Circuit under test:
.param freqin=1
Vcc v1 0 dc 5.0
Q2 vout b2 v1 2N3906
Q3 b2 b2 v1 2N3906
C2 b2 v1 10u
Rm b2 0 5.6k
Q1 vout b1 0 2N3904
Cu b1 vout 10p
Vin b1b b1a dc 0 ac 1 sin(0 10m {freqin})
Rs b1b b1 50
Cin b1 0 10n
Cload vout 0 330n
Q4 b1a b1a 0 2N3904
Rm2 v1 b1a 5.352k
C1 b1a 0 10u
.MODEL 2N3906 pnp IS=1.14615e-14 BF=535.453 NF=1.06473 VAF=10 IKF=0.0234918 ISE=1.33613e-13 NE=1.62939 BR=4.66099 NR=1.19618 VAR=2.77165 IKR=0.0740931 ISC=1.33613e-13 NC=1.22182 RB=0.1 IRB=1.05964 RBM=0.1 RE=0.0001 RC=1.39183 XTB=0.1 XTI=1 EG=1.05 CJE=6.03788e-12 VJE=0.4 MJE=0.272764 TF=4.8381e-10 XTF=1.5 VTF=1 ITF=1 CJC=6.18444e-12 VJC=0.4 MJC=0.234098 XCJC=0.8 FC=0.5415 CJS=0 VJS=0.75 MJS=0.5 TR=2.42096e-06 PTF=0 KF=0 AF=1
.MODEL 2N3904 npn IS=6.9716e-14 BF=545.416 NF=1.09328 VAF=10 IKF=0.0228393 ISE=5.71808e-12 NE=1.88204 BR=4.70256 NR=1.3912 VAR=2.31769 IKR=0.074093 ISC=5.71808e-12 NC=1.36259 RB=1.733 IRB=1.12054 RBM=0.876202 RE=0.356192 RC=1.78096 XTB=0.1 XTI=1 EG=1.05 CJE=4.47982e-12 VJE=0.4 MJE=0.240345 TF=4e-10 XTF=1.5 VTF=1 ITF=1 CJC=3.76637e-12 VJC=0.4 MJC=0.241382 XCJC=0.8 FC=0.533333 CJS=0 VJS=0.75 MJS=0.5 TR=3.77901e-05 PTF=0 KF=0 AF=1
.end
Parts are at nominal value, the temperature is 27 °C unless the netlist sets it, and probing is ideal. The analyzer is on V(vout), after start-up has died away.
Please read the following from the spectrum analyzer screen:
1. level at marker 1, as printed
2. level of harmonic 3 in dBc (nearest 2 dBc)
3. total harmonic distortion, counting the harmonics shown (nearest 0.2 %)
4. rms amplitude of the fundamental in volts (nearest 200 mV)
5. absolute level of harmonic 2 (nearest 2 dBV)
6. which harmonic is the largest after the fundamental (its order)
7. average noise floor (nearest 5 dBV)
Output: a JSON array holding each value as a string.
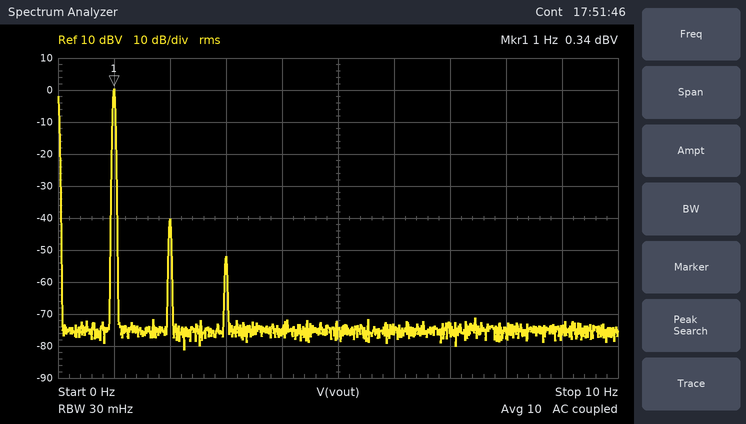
["0.34 dBV", "-52 dBc", "1.0 %", "1.0 V", "-40 dBV", "2", "-75 dBV"]
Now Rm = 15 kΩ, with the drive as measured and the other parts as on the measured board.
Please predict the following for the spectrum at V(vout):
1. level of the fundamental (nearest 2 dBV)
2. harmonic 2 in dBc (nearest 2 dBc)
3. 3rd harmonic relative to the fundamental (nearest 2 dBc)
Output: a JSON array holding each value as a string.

["-36 dBV", "-14 dBc", "-26 dBc"]
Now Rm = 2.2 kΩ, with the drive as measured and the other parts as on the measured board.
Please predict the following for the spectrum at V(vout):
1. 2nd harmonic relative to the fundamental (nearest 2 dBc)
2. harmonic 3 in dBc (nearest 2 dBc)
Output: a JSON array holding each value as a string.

["-10 dBc", "-18 dBc"]
